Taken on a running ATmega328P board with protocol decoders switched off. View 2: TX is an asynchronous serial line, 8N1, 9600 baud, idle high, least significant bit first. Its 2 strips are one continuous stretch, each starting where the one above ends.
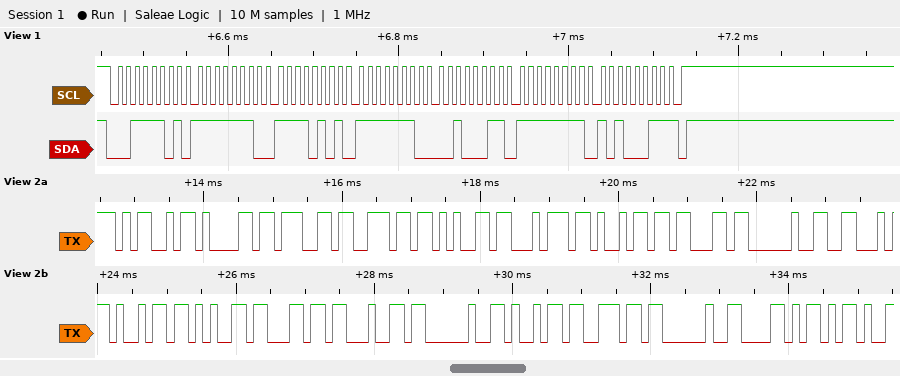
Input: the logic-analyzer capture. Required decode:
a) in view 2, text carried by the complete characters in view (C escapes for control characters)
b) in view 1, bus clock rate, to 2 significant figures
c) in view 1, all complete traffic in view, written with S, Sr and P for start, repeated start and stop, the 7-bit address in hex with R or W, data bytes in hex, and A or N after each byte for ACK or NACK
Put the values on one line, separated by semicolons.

"Magnetic Field in X-"; 100 kHz; S 1ER A FE A F5 A FE A 23 A FF A A3 N P
